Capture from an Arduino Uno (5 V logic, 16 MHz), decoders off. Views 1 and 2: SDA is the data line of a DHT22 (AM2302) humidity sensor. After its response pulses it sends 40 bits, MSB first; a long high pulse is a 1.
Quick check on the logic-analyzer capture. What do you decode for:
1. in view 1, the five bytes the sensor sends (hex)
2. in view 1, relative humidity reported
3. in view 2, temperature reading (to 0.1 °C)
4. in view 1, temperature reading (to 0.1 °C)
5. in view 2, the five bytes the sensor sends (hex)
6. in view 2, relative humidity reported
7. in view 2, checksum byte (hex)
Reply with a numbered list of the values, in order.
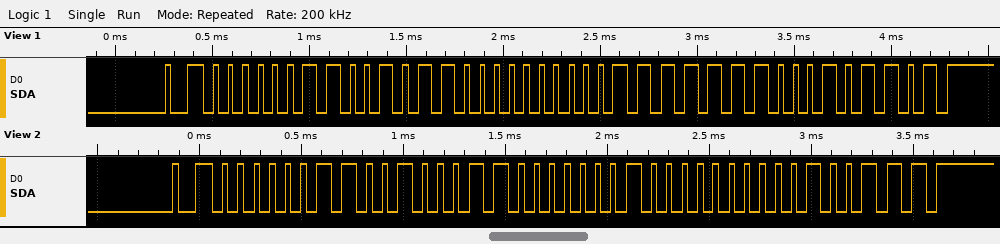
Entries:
1. 03 2C 00 FE 2D
2. 81.2 %
3. 25.6 °C
4. 25.4 °C
5. 03 23 01 00 27
6. 80.3 %
7. 0x27
